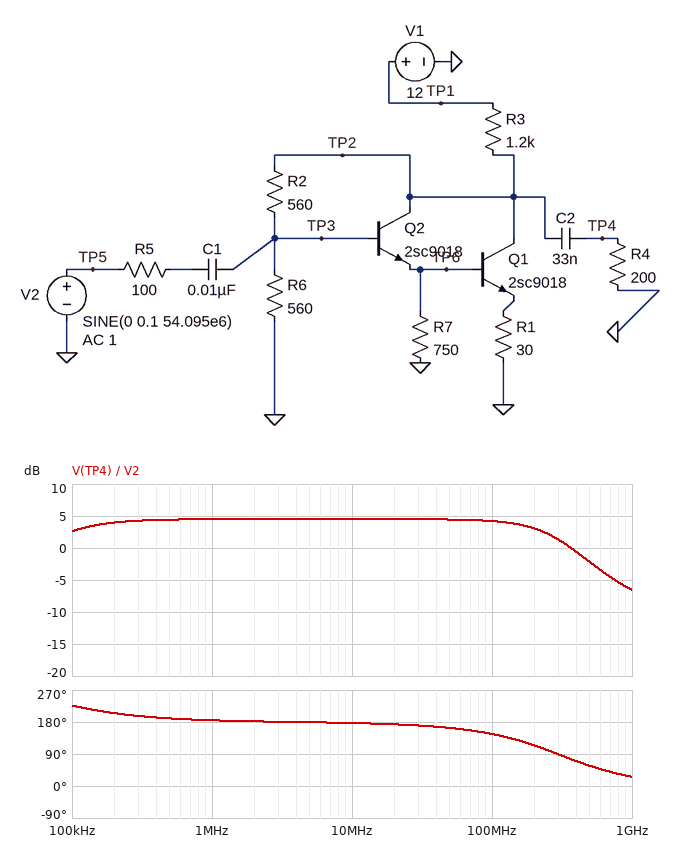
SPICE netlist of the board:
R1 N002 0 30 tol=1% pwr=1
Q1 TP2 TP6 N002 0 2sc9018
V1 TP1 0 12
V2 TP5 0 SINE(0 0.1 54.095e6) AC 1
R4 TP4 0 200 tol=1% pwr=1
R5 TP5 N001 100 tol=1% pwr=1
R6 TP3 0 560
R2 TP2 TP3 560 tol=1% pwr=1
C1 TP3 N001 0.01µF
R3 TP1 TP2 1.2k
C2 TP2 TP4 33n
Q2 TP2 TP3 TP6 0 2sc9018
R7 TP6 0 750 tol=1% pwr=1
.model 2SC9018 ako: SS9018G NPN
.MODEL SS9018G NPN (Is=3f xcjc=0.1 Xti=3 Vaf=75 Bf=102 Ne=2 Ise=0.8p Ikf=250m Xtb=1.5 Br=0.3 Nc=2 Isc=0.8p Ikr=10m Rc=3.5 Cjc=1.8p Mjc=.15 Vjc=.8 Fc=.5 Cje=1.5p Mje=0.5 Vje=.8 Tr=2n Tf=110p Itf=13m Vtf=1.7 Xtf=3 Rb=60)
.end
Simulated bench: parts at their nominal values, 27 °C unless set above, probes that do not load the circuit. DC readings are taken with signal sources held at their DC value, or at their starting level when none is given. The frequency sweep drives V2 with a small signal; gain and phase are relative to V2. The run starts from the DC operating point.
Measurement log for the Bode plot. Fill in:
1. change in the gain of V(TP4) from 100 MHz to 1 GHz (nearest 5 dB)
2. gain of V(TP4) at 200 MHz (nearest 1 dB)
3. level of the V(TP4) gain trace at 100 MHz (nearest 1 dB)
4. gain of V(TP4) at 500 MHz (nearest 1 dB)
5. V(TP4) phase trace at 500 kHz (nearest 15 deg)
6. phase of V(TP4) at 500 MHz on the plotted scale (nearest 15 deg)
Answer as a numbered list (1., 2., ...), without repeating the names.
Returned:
1. -10 dB
2. 3 dB
3. 4 dB
4. -2 dB
5. 195 deg
6. 60 deg
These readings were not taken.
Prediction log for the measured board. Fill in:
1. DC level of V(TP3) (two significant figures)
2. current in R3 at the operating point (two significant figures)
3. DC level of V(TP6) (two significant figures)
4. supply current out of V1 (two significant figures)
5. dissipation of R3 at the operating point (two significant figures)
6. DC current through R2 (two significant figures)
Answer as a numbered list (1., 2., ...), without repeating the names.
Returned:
1. 1.5 V
2. 7.5 mA
3. 830 mV
4. 7.5 mA
5. 67 mW
6. 2.7 mA
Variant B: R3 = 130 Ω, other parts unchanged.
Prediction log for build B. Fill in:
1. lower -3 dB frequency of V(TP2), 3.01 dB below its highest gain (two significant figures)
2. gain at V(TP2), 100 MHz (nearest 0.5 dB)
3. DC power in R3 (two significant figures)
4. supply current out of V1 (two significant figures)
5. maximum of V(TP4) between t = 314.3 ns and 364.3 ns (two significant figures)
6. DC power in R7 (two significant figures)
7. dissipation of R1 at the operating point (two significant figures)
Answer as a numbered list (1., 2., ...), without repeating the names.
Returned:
1. 62 kHz
2. 1.5 dB
3. 320 mW
4. 49 mA
5. 120 mV
6. 5.7 mW
7. 52 mW
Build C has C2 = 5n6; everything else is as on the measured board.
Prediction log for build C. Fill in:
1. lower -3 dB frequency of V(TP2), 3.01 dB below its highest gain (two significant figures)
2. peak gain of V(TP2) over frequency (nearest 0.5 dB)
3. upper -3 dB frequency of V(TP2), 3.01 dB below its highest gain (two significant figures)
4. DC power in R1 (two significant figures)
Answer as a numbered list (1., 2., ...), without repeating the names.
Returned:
1. 52 kHz
2. 5.5 dB
3. 220 MHz
4. 400 µW
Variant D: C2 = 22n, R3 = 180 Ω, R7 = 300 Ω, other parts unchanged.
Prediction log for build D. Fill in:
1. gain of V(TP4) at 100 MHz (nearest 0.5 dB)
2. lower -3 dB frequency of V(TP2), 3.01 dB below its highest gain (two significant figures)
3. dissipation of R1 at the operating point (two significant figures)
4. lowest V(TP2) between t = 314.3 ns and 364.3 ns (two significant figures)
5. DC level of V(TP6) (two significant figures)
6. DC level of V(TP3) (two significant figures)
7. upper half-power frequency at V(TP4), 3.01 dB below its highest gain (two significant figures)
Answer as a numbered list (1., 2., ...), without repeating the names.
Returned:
1. 3.0 dB
2. 62 kHz
3. 26 mW
4. 4.7 V
5. 1.7 V
6. 2.4 V
7. 270 MHz
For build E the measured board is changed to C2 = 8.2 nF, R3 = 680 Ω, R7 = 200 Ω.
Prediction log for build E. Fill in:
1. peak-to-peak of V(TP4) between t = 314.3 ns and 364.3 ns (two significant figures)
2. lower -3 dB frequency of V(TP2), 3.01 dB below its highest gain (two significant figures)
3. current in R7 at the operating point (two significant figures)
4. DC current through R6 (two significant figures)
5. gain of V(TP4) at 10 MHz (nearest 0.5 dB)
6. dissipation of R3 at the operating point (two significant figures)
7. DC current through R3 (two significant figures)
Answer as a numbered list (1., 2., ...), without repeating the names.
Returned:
1. 360 mV
2. 52 kHz
3. 4.5 mA
4. 2.9 mA
5. 5.0 dB
6. 110 mW
7. 13 mA
